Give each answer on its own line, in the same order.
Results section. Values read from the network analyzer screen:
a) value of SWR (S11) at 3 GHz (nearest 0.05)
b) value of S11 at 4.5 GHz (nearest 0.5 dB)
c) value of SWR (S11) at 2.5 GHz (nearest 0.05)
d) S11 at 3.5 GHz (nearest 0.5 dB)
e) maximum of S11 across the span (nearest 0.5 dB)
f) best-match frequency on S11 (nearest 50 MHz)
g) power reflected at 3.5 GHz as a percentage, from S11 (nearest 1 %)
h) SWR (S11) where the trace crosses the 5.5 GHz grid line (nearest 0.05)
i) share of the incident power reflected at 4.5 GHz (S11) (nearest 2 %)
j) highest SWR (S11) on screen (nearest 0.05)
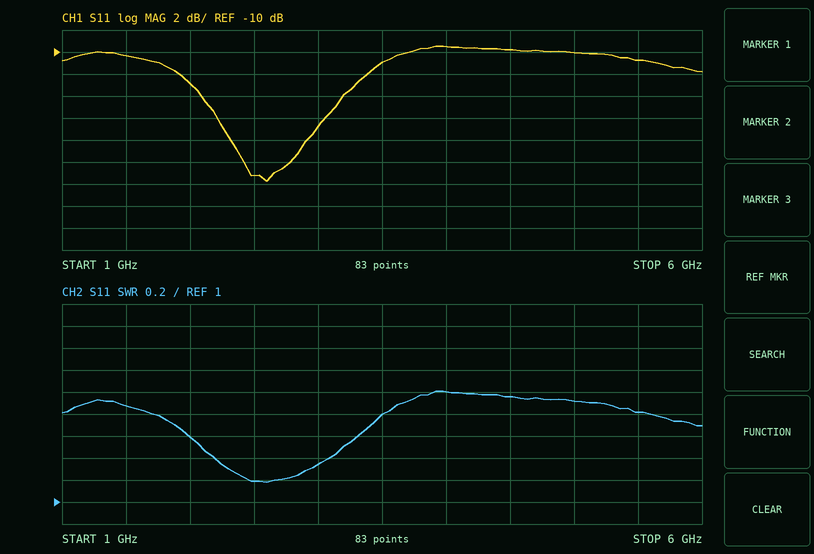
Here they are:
1.35
-10.0 dB
1.20
-11.0 dB
-9.5 dB
2.60 GHz
8 %
1.80
10 %
2.00
